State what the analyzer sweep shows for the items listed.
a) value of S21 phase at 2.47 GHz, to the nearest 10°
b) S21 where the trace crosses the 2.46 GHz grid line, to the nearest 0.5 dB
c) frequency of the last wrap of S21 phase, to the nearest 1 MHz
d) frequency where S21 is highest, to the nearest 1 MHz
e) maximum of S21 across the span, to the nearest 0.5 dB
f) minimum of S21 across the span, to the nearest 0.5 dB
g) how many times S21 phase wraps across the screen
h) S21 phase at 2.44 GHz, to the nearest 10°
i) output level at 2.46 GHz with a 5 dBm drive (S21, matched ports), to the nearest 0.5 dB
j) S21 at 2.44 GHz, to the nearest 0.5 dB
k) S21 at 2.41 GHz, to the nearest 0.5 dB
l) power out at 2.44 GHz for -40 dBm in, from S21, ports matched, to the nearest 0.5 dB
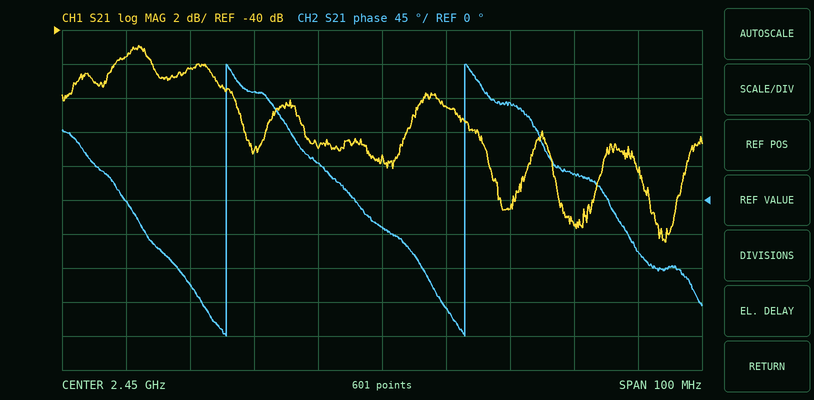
130°
-44.5 dB
2.463 GHz
2.412 GHz
-41.0 dB
-52.5 dB
2
50°
-39.5 dBm
-47.0 dB
-41.5 dB
-87.0 dBm
